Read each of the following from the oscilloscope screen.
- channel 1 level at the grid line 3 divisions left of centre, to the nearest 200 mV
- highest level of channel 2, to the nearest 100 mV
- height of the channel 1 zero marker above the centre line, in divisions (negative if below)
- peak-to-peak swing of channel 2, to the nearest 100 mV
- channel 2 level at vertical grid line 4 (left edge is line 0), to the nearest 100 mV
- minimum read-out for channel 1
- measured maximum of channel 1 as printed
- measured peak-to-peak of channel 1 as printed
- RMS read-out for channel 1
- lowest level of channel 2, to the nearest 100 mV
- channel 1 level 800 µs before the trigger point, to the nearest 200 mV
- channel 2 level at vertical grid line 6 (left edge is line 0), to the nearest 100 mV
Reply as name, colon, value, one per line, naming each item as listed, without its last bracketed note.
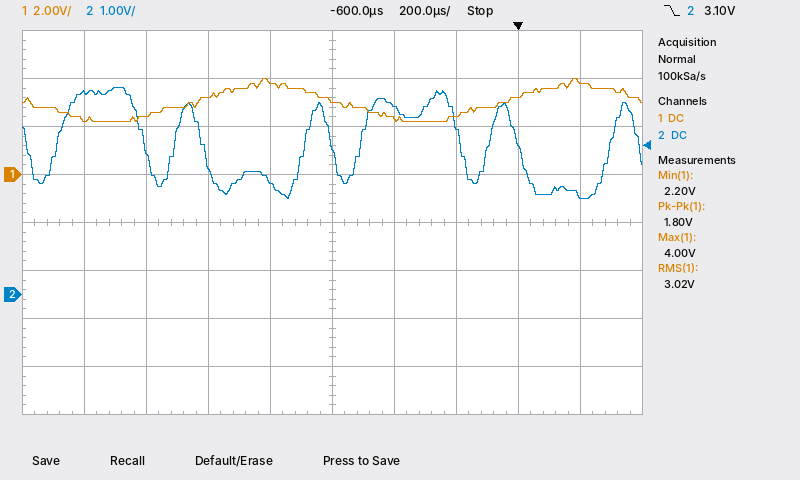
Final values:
channel 1 level at the grid line 3 divisions left of centre, to the nearest 200 mV: 2.4 V
highest level of channel 2, to the nearest 100 mV: 4.3 V
height of the channel 1 zero marker above the centre line, in divisions: +1.0 div
peak-to-peak swing of channel 2, to the nearest 100 mV: 2.3 V
channel 2 level at vertical grid line 4 (left edge is line 0), to the nearest 100 mV: 2.4 V
minimum read-out for channel 1: 2.20 V
measured maximum of channel 1 as printed: 4.00 V
measured peak-to-peak of channel 1 as printed: 1.80 V
RMS read-out for channel 1: 3.02 V
lowest level of channel 2, to the nearest 100 mV: 2.0 V
channel 1 level 800 µs before the trigger point, to the nearest 200 mV: 3.8 V
channel 2 level at vertical grid line 6 (left edge is line 0), to the nearest 100 mV: 3.9 V
